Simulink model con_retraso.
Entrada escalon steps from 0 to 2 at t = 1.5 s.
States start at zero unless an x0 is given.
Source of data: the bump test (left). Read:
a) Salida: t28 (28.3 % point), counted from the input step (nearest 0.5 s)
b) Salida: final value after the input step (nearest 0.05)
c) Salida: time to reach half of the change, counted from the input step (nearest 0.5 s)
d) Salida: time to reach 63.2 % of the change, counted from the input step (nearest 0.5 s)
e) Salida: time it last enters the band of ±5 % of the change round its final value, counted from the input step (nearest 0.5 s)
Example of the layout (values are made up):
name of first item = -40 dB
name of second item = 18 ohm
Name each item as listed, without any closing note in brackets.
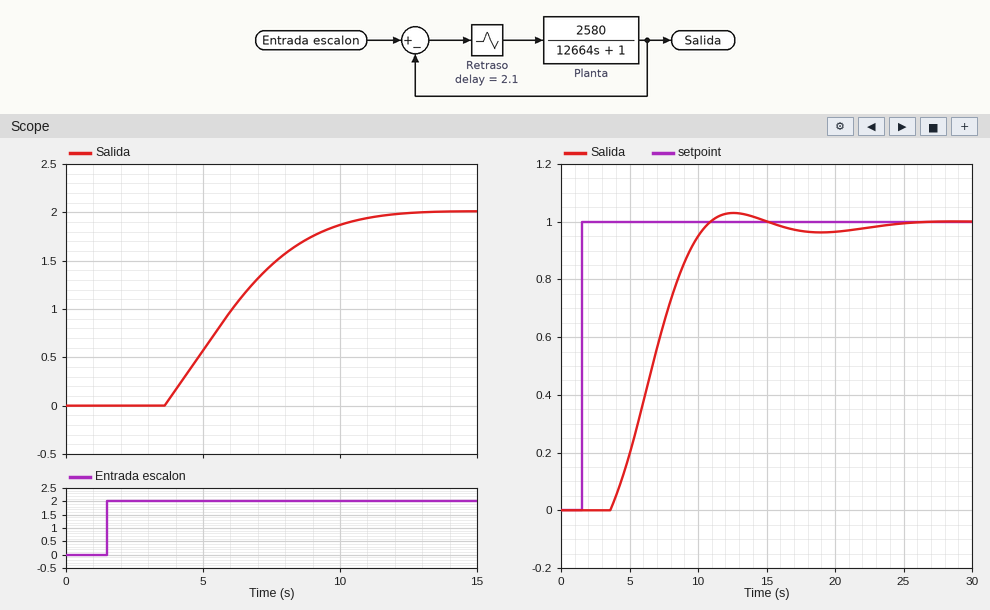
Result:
Salida: t28 (28.3 % point), counted from the input step = 3.5 s
Salida: final value after the input step = 2.00
Salida: time to reach half of the change, counted from the input step = 4.5 s
Salida: time to reach 63.2 % of the change, counted from the input step = 5.5 s
Salida: time it last enters the band of ±5 % of the change round its final value, counted from the input step = 9.0 s
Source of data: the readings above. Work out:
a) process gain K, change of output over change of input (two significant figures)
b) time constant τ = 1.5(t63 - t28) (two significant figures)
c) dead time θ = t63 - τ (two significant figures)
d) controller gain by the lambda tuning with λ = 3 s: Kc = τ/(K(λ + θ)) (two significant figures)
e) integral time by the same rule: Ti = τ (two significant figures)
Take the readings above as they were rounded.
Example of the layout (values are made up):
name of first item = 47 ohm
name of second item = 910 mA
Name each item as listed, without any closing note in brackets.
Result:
process gain K, change of output over change of input = 1.0
time constant τ = 1.5(t63 - t28) = 3.0 s
dead time θ = t63 - τ = 2.5 s
controller gain by the lambda tuning with λ = 3 s: Kc = τ/(K(λ + θ)) = 0.55
integral time by the same rule: Ti = τ = 3.0 s
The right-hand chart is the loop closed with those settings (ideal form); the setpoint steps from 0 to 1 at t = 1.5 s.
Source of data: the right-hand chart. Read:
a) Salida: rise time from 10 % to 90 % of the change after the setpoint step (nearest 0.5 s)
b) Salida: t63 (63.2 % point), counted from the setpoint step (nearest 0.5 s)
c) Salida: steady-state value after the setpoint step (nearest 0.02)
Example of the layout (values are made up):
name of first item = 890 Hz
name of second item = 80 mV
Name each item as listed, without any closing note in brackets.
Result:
Salida: rise time from 10 % to 90 % of the change after the setpoint step = 5.0 s
Salida: t63 (63.2 % point), counted from the setpoint step = 6.0 s
Salida: steady-state value after the setpoint step = 1.00
